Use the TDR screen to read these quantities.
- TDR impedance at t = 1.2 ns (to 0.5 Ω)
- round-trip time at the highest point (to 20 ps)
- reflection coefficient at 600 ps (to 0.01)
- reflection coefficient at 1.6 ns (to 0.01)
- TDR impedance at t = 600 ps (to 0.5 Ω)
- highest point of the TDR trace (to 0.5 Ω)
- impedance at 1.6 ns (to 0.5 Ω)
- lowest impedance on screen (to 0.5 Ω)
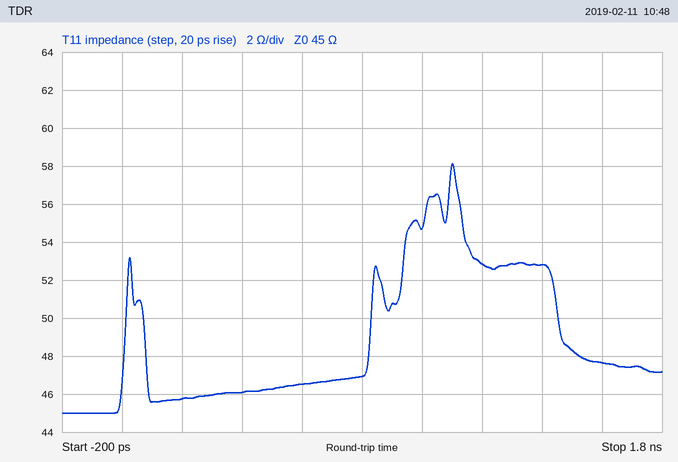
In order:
53.0 Ω
1.10 ns
+0.02
+0.03
46.5 Ω
58.0 Ω
47.5 Ω
45.0 Ω
